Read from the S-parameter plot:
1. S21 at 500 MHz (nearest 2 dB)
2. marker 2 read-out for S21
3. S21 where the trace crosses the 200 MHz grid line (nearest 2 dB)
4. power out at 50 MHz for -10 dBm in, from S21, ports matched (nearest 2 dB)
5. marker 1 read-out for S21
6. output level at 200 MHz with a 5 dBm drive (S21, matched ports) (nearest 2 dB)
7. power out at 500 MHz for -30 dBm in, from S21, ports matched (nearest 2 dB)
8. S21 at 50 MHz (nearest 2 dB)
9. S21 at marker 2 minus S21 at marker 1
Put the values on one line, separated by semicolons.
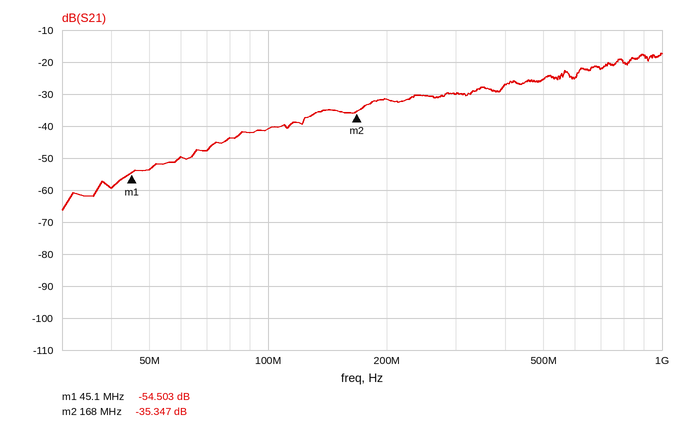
-26 dB; -35.347 dB; -32 dB; -64 dBm; -54.503 dB; -26 dBm; -56 dBm; -54 dB; 19.156 dB
